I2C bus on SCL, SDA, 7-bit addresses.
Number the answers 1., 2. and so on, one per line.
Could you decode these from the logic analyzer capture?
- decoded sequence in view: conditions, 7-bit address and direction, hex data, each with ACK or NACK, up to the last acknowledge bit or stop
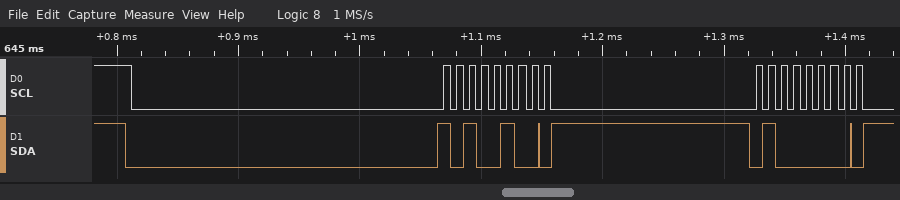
1. start, address 52 write ACK, 40 ACK
